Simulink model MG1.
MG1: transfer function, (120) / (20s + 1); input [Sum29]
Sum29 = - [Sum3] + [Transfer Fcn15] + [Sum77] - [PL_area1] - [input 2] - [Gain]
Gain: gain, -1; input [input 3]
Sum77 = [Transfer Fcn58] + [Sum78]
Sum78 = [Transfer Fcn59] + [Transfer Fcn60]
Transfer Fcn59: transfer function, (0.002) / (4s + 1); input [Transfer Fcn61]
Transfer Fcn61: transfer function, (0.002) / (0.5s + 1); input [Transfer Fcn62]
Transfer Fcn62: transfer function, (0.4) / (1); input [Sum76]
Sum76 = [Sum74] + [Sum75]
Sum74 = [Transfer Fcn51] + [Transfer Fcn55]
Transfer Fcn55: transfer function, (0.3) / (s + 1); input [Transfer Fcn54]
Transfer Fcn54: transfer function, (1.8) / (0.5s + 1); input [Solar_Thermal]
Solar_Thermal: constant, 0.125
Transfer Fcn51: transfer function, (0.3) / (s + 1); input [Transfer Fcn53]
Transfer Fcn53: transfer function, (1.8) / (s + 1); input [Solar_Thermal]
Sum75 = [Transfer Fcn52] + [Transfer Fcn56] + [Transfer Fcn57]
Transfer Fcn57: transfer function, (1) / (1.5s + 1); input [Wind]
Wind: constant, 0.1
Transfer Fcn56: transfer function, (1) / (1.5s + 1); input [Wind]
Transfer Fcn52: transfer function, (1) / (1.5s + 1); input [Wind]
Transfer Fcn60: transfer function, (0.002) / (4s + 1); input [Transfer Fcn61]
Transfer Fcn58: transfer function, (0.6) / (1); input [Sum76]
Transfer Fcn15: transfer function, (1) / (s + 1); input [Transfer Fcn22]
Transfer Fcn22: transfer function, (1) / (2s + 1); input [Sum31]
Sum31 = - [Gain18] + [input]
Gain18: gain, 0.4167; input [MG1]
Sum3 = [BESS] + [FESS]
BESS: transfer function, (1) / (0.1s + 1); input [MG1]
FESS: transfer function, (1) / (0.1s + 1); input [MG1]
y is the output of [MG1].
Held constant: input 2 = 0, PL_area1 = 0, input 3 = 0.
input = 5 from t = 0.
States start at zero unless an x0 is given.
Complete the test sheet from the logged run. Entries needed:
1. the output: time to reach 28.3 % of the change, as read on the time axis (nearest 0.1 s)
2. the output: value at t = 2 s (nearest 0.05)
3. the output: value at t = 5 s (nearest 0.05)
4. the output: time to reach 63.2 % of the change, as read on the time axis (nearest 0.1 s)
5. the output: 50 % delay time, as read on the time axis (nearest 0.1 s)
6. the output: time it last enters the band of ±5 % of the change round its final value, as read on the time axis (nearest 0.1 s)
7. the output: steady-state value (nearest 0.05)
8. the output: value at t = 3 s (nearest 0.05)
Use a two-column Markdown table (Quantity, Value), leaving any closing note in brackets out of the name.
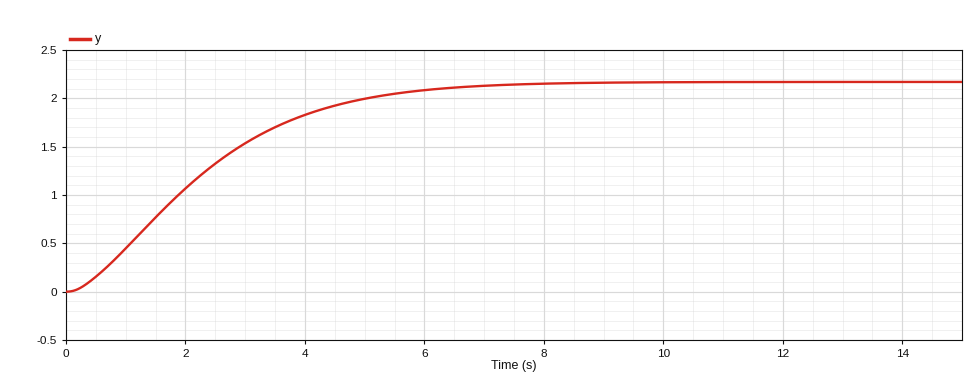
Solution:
| Quantity | Value |
|---|---|
| the output: time to reach 28.3 % of the change, as read on the time axis | 1.3 s |
| the output: value at t = 2 s | 1.05 |
| the output: value at t = 5 s | 2.00 |
| the output: time to reach 63.2 % of the change, as read on the time axis | 2.6 s |
| the output: 50 % delay time, as read on the time axis | 2.0 s |
| the output: time it last enters the band of ±5 % of the change round its final value, as read on the time axis | 5.7 s |
| the output: steady-state value | 2.15 |
| the output: value at t = 3 s | 1.55 |
